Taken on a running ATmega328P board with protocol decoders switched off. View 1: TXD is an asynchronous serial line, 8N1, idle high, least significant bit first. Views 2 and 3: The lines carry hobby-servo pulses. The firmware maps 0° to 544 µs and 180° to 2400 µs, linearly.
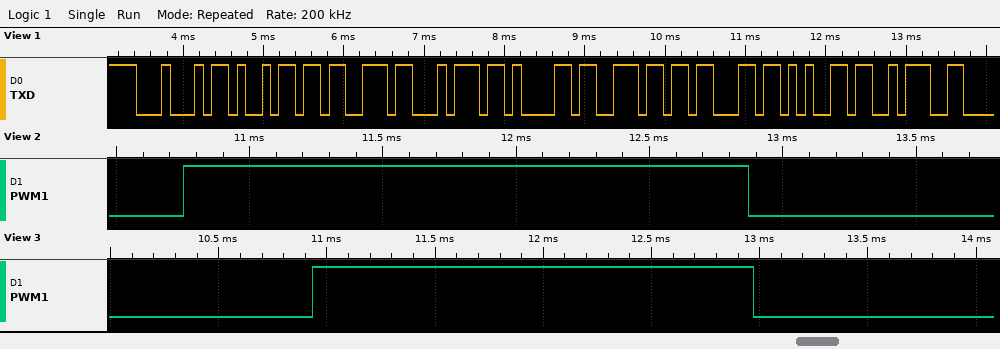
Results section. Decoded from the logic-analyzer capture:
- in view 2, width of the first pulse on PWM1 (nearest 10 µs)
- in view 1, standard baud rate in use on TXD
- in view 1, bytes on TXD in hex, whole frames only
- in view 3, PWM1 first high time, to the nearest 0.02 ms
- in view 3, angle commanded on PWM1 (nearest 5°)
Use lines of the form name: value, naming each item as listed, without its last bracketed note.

in view 2, width of the first pulse on PWM1: 2120 µs
in view 1, standard baud rate in use on TXD: 9600 baud
in view 1, bytes on TXD in hex, whole frames only: 44 69 73 74 61 6E 63 65 3A
in view 3, PWM1 first high time, to the nearest 0.02 ms: 2.04 ms
in view 3, angle commanded on PWM1: 145°
